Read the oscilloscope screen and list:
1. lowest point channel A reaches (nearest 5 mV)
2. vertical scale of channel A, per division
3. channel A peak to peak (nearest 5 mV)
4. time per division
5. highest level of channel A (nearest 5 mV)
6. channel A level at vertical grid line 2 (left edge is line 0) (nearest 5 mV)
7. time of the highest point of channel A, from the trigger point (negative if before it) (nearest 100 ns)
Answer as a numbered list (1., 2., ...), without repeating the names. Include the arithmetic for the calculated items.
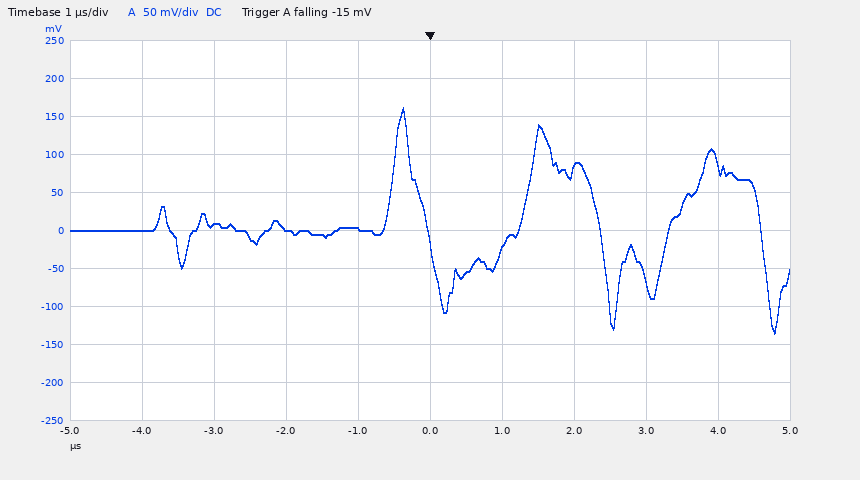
1. -135 mV
2. 50 mV
3. 160 mV − (-135 mV) = 295 mV
4. 1 µs
5. 160 mV
6. 5 mV
7. -400 ns
